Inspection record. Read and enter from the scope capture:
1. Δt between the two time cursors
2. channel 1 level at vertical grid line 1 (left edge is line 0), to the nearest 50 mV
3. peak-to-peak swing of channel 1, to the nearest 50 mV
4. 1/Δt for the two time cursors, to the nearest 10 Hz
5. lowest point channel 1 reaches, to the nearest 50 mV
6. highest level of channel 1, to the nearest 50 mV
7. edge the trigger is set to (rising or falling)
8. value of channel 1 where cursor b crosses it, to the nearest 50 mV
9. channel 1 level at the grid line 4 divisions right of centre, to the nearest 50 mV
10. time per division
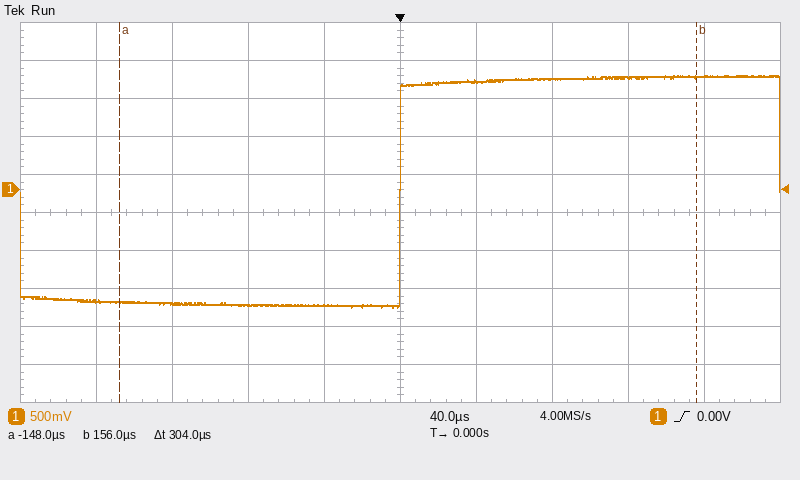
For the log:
304 µs
-1.45 V
3.05 V
3.29 kHz
-1.55 V
1.50 V
rising
1.50 V
1.50 V
40 µs
